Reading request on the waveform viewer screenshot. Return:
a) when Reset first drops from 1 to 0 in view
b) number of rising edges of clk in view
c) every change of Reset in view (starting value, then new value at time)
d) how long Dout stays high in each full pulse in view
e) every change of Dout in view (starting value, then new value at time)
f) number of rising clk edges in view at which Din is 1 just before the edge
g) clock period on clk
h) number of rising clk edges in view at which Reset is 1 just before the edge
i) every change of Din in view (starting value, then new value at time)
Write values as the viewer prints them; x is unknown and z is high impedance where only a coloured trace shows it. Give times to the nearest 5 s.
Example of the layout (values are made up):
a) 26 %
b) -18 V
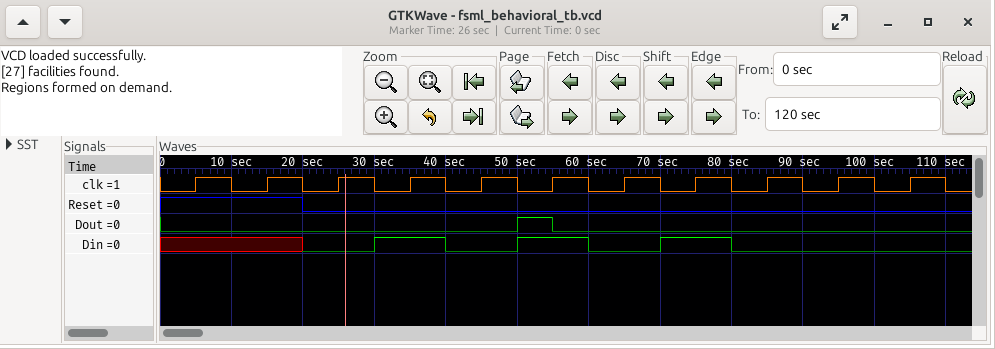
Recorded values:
a) 20 s
b) 11
c) 1, 0 at 20 s
d) 5 s
e) 0, 1 at 50 s, 0 at 55 s
f) 3
g) 10 s
h) 2
i) x, 0 at 20 s, 1 at 30 s, 0 at 40 s, 1 at 50 s, 0 at 60 s, 1 at 70 s, 0 at 80 s
